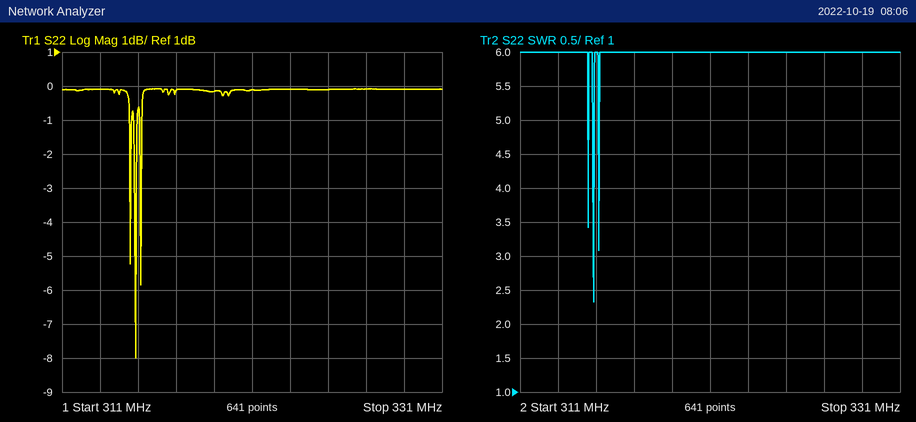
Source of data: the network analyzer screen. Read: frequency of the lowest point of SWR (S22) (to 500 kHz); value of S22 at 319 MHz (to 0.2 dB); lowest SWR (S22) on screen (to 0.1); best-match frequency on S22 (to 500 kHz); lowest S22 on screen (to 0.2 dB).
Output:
315.0 MHz
-0.2 dB
2.3
315.0 MHz
-8.0 dB
